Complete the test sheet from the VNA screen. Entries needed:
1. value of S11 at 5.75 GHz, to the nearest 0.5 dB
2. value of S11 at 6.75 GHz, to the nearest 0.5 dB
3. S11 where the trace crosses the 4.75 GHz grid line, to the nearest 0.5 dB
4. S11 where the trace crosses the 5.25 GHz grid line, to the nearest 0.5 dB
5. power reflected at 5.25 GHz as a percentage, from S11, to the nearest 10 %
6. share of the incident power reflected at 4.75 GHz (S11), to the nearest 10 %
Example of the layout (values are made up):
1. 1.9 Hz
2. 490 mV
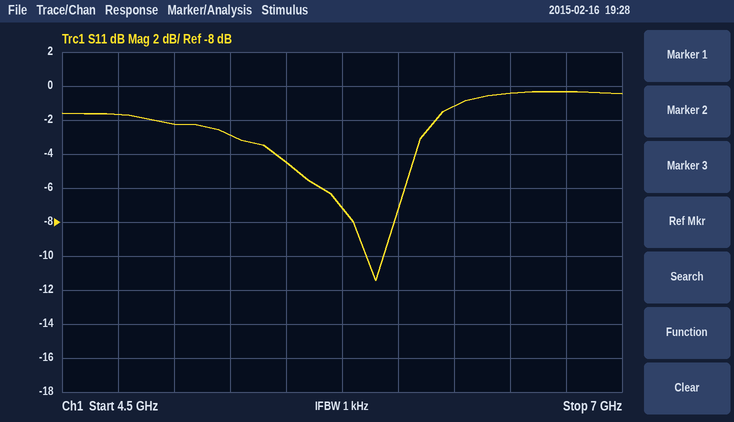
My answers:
1. -7.0 dB
2. -0.5 dB
3. -1.5 dB
4. -3.0 dB
5. 50 %
6. 70 %
